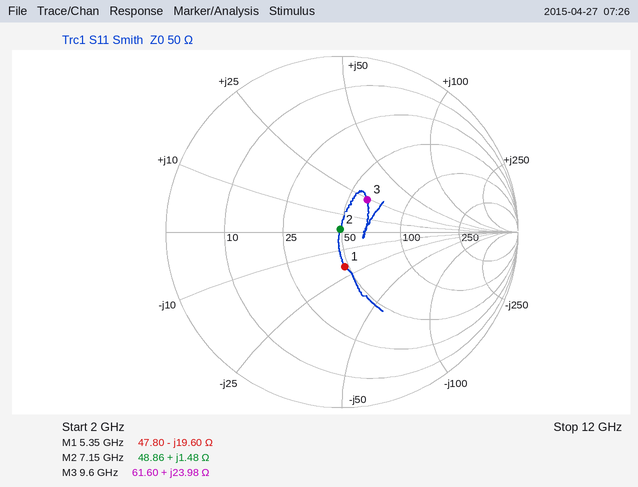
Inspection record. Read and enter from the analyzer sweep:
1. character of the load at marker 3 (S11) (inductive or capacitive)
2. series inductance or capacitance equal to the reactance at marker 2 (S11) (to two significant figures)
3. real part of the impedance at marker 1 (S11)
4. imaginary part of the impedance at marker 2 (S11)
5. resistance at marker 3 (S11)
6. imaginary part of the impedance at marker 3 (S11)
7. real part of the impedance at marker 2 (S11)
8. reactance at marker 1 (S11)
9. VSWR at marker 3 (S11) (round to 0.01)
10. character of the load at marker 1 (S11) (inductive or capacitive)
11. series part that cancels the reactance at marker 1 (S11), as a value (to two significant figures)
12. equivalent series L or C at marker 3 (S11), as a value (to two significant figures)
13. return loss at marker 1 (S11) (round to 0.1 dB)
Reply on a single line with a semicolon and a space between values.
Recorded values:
inductive; 33 pH; 47.80 Ω; +1.48 Ω; 61.60 Ω; +23.98 Ω; 48.86 Ω; -19.60 Ω; 1.61; capacitive; 580 pH; 400 pH; 14.1 dB
